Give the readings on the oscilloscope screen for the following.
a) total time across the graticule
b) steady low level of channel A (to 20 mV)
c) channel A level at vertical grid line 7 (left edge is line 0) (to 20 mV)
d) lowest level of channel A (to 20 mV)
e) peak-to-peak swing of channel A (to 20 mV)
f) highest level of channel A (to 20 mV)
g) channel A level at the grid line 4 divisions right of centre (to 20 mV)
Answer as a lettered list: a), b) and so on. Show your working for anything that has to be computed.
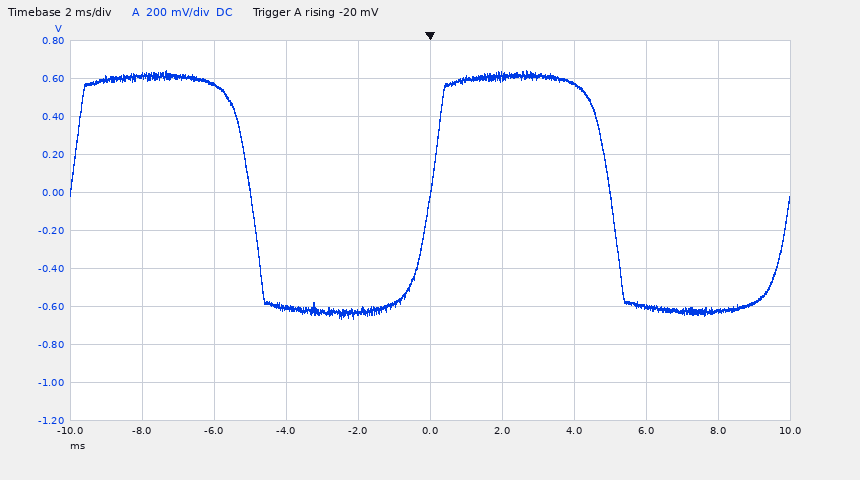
a) 20 ms
b) -620 mV
c) 580 mV
d) -660 mV
e) 640 mV − (-660 mV) = 1.30 V
f) 640 mV
g) -620 mV
